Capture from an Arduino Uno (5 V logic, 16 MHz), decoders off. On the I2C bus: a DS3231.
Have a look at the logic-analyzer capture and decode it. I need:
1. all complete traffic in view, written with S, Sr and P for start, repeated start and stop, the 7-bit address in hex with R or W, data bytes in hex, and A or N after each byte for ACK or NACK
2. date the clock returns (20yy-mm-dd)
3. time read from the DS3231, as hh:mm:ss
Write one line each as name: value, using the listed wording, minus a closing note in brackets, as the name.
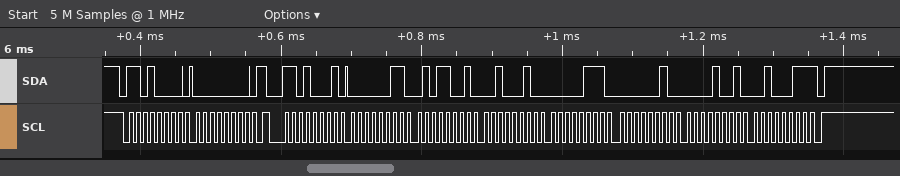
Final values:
all complete traffic in view, written with S, Sr and P for start, repeated start and stop, the 7-bit address in hex with R or W, data bytes in hex, and A or N after each byte for ACK or NACK: S 68W A 00 A Sr 68R A 03 A 59 A 22 A 07 A 02 A 09 A 23 N P
date the clock returns: 2023-09-02
time read from the DS3231, as hh:mm:ss: 22:59:03
